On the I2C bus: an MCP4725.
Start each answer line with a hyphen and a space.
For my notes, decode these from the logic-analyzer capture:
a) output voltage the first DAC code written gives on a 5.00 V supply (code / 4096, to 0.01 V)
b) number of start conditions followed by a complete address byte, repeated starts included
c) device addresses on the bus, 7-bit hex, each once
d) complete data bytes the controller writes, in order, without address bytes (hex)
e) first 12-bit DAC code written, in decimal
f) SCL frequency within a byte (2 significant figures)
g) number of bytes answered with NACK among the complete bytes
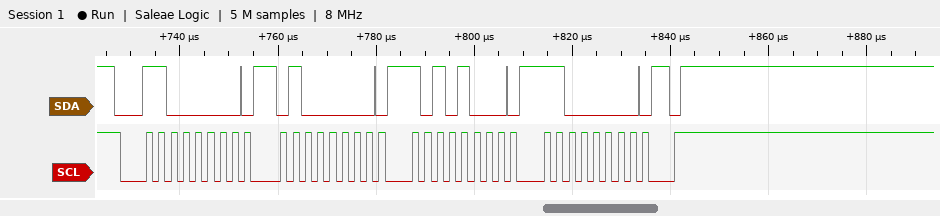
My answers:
- 3.30 V
- 1
- 0x60
- 40 A8 C0
- 2700
- 400 kHz
- 0
